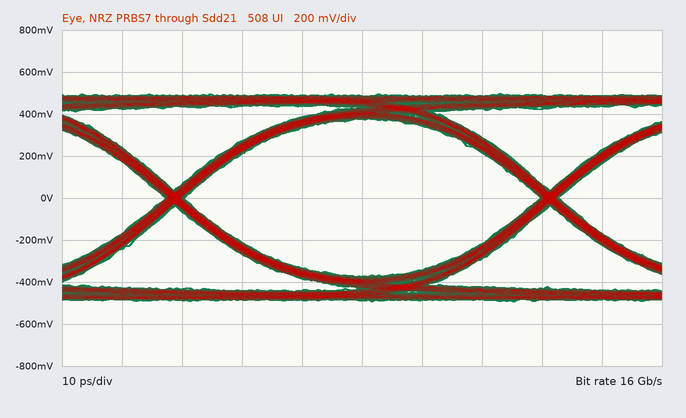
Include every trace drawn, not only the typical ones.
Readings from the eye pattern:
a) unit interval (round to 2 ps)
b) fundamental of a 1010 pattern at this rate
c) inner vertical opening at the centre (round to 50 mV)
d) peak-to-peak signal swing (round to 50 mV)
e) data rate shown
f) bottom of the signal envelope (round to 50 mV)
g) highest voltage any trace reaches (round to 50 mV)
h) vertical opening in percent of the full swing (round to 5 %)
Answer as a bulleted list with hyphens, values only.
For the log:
- 62 ps
- 8 GHz
- 750 mV
- 1.00 V
- 16 Gb/s
- -500 mV
- 500 mV
- 75 %
